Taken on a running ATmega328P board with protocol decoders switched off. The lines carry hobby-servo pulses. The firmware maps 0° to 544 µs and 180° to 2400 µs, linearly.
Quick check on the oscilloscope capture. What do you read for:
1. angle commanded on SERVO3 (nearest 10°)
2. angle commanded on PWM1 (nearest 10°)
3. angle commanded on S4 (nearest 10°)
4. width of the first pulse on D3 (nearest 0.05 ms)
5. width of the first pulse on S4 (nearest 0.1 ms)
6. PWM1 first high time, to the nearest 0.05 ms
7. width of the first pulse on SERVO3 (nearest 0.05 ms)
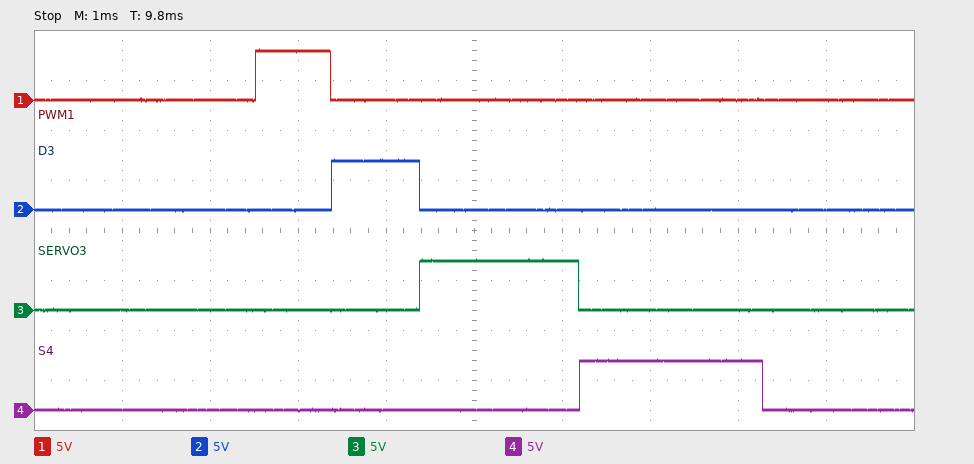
120°
30°
150°
1.00 ms
2.1 ms
0.85 ms
1.80 ms
